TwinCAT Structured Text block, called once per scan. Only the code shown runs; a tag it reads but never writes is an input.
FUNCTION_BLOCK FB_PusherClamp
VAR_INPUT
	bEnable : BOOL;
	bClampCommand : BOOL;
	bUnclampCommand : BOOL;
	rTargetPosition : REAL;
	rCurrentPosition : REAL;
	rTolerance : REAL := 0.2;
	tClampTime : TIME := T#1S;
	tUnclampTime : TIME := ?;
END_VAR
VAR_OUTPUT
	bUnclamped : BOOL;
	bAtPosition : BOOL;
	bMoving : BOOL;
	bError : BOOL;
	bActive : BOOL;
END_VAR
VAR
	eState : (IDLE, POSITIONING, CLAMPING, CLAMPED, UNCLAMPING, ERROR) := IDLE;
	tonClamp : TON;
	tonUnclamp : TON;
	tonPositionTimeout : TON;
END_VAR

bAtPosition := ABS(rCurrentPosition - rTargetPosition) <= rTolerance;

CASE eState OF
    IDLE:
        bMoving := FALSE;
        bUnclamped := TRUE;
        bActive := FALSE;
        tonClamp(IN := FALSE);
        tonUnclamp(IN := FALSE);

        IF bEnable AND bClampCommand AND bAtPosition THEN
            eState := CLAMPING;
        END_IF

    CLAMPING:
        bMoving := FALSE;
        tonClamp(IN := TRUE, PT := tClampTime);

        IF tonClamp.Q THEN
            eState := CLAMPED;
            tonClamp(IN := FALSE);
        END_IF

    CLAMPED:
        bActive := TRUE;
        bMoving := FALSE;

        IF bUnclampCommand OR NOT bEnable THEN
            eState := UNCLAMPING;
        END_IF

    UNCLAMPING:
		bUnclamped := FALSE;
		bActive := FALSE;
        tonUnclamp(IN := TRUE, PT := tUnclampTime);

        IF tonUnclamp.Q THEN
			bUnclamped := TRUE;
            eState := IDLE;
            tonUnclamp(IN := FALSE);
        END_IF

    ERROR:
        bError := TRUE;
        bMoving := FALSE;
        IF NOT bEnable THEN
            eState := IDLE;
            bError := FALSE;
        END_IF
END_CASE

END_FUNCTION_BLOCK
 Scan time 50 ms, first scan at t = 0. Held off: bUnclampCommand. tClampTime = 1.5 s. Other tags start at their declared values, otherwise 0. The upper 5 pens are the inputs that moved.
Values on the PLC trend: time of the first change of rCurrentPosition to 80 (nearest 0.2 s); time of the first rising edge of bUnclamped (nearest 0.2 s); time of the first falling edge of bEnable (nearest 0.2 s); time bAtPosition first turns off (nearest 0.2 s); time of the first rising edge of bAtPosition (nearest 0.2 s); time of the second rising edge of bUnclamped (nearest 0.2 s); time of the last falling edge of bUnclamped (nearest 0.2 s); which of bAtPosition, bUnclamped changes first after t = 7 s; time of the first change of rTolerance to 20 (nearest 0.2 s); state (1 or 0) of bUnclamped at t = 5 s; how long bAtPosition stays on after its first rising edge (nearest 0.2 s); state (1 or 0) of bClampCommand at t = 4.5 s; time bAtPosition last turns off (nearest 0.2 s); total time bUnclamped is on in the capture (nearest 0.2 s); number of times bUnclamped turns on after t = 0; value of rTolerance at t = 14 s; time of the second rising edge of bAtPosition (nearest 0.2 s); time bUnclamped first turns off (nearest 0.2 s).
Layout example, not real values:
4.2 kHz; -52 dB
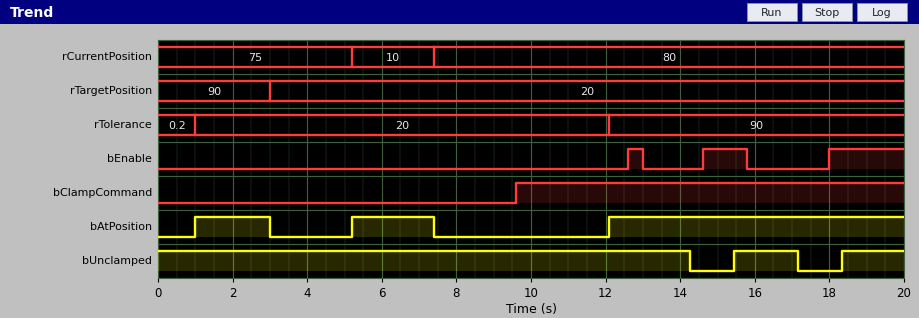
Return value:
7.4 s; 15.4 s; 13.0 s; 3.0 s; 1.0 s; 18.4 s; 17.2 s; bAtPosition; 1.0 s; 1; 2.0 s; 0; 7.4 s; 17.6 s; 2; 90; 5.2 s; 14.2 s
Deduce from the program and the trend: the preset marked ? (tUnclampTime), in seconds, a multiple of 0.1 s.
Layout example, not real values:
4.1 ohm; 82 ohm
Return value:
1.2 s
